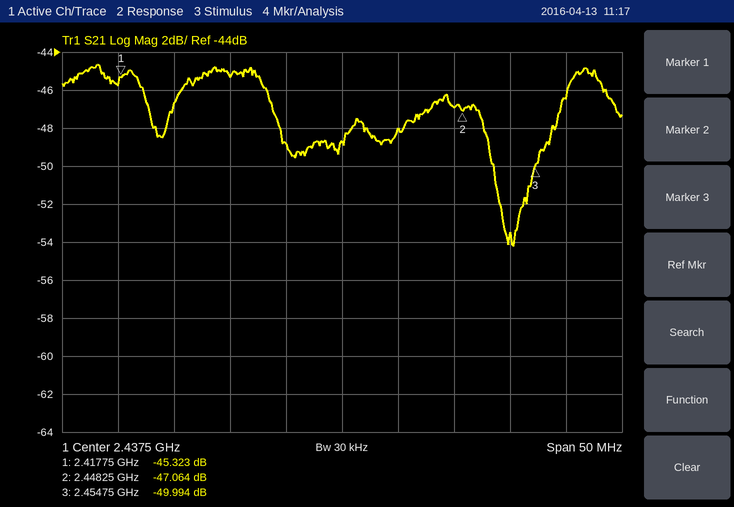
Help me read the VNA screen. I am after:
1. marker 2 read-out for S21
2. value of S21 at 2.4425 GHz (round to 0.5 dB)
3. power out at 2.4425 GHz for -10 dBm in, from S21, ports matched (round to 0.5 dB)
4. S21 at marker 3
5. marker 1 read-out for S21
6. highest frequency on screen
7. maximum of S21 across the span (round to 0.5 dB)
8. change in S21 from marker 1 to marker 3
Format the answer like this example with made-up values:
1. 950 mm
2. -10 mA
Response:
1. -47.064 dB
2. -48.0 dB
3. -58.0 dBm
4. -49.994 dB
5. -45.323 dB
6. 2.4625 GHz
7. -44.5 dB
8. -4.671 dB
